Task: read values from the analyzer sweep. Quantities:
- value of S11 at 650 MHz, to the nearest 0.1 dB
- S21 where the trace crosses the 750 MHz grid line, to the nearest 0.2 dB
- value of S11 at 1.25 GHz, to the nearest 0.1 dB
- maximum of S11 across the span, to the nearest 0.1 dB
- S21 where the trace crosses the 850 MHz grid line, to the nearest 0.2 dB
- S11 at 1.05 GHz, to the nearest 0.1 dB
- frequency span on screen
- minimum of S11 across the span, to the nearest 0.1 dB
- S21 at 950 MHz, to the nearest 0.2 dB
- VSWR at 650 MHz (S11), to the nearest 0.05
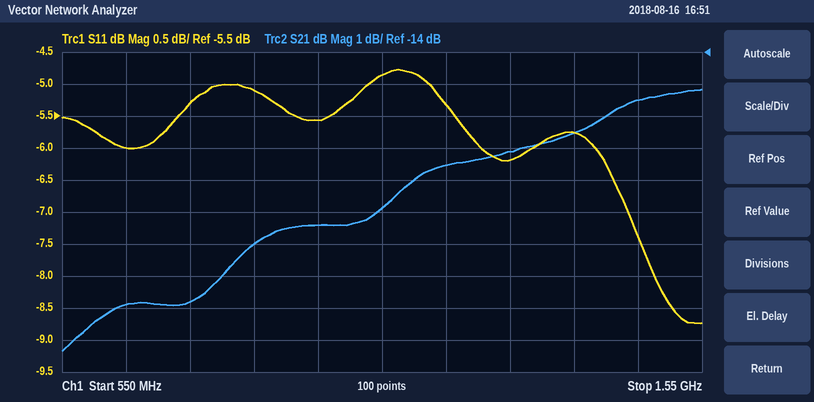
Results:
-6.0 dB
-21.8 dB
-6.2 dB
-4.8 dB
-20.0 dB
-4.9 dB
1 GHz
-8.7 dB
-19.4 dB
3.00
